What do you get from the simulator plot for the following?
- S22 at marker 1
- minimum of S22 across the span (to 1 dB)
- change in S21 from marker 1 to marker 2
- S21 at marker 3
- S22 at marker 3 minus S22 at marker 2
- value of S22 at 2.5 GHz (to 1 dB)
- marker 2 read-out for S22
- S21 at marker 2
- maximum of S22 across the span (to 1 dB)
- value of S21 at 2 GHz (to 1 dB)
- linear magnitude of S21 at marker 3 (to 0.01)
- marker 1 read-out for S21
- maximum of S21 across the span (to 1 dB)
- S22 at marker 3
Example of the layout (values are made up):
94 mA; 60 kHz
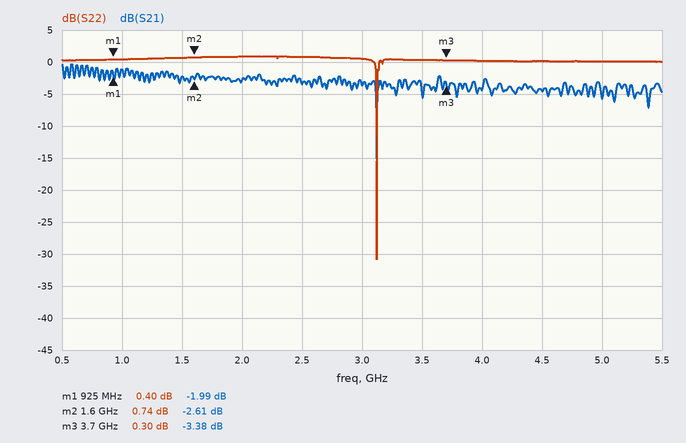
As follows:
0.40 dB; -31 dB; -0.62 dB; -3.38 dB; -0.44 dB; 1 dB; 0.74 dB; -2.61 dB; 1 dB; -3 dB; 0.68; -1.99 dB; 0 dB; 0.30 dB
